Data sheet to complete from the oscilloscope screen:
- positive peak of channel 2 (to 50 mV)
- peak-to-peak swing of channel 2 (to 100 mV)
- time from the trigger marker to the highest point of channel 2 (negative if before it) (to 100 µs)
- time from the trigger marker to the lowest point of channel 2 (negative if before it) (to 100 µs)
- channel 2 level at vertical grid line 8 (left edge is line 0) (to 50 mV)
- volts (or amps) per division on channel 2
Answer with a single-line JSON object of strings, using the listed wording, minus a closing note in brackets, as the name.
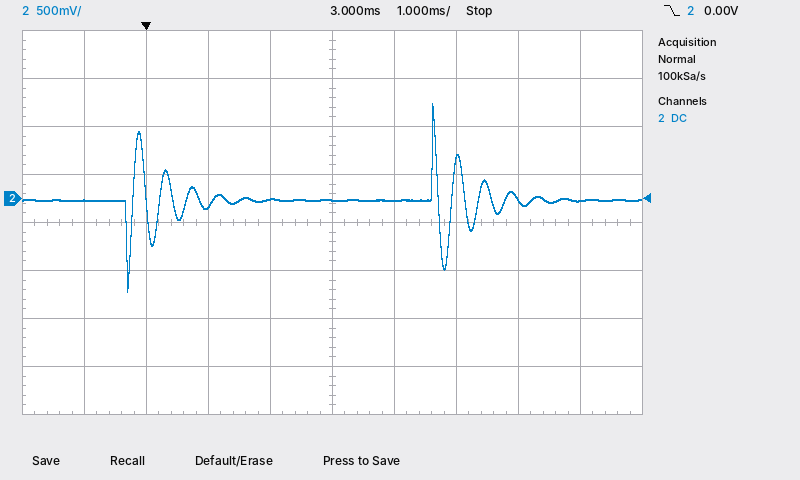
{"positive peak of channel 2": "1.00 V", "peak-to-peak swing of channel 2": "2.00 V", "time from the trigger marker to the highest point of channel 2 (negative if before it)": "+4.6 ms", "time from the trigger marker to the lowest point of channel 2 (negative if before it)": "-300 µs", "channel 2 level at vertical grid line 8 (left edge is line 0)": "0 mV", "volts (or amps) per division on channel 2": "500 mV"}
